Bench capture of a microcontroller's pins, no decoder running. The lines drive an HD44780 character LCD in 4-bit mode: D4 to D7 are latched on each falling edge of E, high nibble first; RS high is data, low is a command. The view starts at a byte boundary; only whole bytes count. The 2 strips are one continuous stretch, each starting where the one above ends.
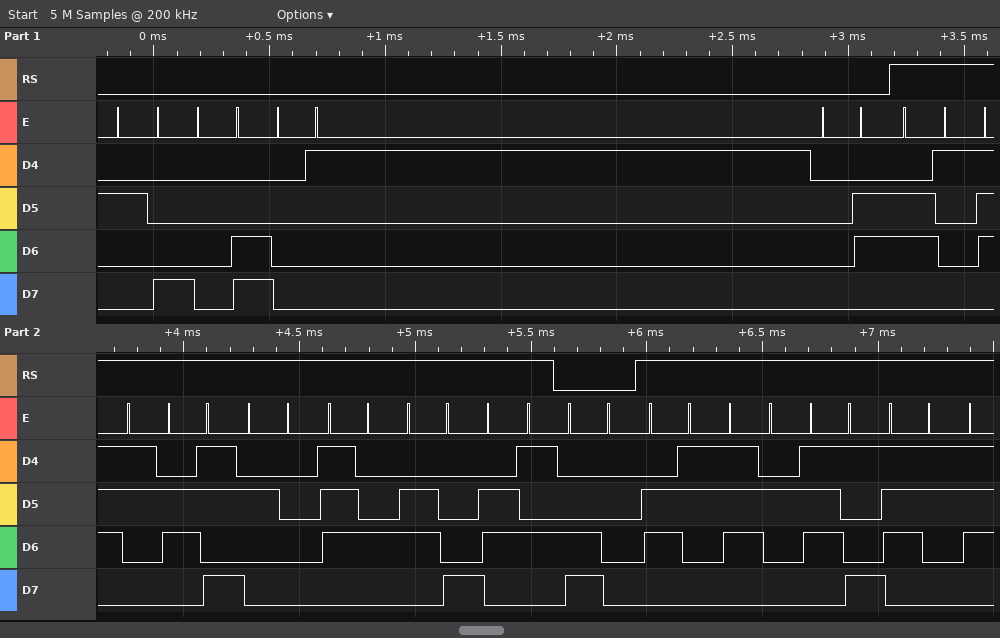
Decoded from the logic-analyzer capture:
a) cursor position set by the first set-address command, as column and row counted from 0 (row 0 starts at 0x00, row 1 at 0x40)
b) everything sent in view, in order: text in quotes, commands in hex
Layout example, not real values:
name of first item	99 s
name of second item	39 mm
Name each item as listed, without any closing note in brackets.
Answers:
cursor position set by the first set-address command, as column and row counted from 0	column 0, row 1
everything sent in view, in order: text in quotes, commands in hex	0x28 0x0C 0x01 0x06 "ask the" 0xC0 "crys"
